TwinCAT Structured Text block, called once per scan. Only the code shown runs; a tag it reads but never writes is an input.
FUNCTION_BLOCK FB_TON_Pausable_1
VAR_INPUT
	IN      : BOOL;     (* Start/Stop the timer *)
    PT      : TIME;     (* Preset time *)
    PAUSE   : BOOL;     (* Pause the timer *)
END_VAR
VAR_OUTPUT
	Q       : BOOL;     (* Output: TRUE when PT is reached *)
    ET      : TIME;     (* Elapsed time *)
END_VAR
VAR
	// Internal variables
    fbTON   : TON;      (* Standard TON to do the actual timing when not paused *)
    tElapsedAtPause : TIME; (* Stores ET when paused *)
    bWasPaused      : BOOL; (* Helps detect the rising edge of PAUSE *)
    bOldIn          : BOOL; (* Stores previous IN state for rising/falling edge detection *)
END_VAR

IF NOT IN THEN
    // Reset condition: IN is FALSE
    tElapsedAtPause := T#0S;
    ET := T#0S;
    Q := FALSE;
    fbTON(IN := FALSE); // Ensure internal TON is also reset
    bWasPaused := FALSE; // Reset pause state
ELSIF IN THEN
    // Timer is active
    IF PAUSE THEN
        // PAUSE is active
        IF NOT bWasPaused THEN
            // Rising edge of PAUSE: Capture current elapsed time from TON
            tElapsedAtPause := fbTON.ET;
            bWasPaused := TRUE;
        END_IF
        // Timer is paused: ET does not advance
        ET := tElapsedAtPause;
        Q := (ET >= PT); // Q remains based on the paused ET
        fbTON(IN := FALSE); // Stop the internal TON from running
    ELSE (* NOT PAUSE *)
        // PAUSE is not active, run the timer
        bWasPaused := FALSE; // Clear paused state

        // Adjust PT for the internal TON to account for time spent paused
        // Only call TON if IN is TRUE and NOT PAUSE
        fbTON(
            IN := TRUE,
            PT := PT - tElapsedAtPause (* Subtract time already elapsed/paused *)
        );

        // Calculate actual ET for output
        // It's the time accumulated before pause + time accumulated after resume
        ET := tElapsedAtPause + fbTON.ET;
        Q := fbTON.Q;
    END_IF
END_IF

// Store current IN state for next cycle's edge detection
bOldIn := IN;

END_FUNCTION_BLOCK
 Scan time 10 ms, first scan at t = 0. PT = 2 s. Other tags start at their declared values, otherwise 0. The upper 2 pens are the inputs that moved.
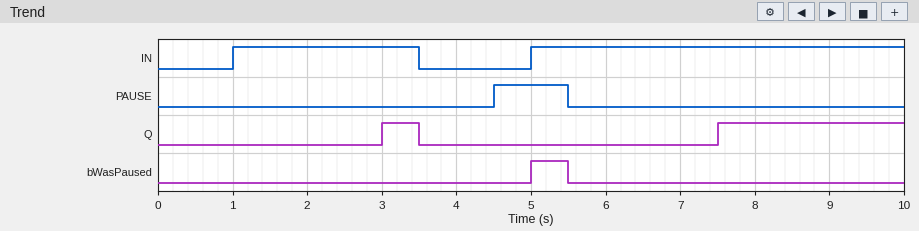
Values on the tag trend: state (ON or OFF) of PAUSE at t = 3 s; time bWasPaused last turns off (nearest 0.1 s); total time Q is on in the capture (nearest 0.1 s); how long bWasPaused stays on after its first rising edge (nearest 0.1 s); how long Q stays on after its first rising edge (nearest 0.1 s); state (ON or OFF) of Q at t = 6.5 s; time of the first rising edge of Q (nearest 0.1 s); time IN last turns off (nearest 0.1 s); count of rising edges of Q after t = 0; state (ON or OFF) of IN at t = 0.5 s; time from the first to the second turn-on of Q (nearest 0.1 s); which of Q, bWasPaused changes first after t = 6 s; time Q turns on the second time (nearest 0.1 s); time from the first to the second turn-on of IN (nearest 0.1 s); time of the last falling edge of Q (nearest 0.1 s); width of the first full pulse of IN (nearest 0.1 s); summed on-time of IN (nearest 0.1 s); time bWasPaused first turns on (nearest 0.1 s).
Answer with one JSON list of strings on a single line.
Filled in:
["OFF", "5.5 s", "3.0 s", "0.5 s", "0.5 s", "OFF", "3.0 s", "3.5 s", "2", "OFF", "4.5 s", "Q", "7.5 s", "4.0 s", "3.5 s", "2.5 s", "7.5 s", "5.0 s"]
